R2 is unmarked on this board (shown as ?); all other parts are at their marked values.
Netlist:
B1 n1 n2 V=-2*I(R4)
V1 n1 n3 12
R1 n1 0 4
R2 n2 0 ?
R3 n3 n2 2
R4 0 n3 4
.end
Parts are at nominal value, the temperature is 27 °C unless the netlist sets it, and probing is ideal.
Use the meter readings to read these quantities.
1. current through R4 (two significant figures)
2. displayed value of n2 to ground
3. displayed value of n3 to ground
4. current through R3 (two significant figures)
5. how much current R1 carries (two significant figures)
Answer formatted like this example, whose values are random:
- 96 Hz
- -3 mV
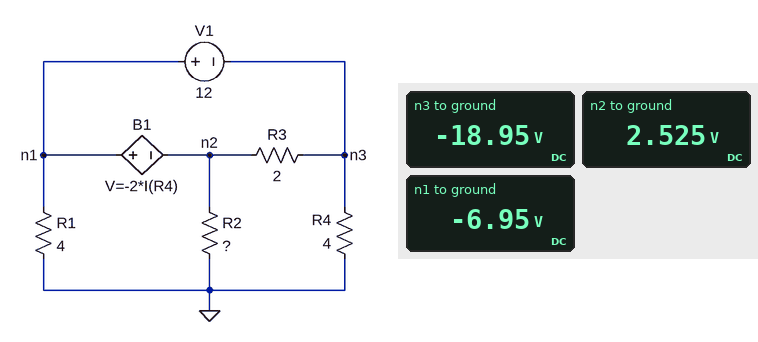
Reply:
- 4.7 A
- 2.525 V
- -18.95 V
- 11 A
- 1.7 A
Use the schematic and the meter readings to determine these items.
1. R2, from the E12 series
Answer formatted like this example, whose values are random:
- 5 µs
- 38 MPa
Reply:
- 0.39 Ω
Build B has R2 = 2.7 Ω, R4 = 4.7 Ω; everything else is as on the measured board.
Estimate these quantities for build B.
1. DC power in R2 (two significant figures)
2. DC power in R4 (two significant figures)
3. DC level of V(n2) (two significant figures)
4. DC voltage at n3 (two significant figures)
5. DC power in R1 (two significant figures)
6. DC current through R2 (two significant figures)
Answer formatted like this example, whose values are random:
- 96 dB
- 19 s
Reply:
- 12 W
- 26 W
- 5.7 V
- -11 V
- 240 mW
- 2.1 A
